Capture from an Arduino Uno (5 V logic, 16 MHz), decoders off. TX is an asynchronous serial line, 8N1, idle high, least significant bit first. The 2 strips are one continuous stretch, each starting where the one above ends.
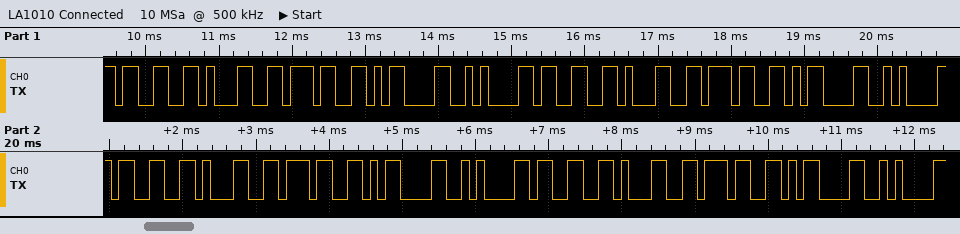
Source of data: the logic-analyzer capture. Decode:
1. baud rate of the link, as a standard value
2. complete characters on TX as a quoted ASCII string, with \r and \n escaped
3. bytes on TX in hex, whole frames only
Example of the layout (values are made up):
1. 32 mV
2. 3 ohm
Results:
1. 9600 baud
2. "317\r\n317\r\n317\r\n317\r\n"
3. 0x33 0x31 0x37 0x0D 0x0A 0x33 0x31 0x37 0x0D 0x0A 0x33 0x31 0x37 0x0D 0x0A 0x33 0x31 0x37 0x0D 0x0A
